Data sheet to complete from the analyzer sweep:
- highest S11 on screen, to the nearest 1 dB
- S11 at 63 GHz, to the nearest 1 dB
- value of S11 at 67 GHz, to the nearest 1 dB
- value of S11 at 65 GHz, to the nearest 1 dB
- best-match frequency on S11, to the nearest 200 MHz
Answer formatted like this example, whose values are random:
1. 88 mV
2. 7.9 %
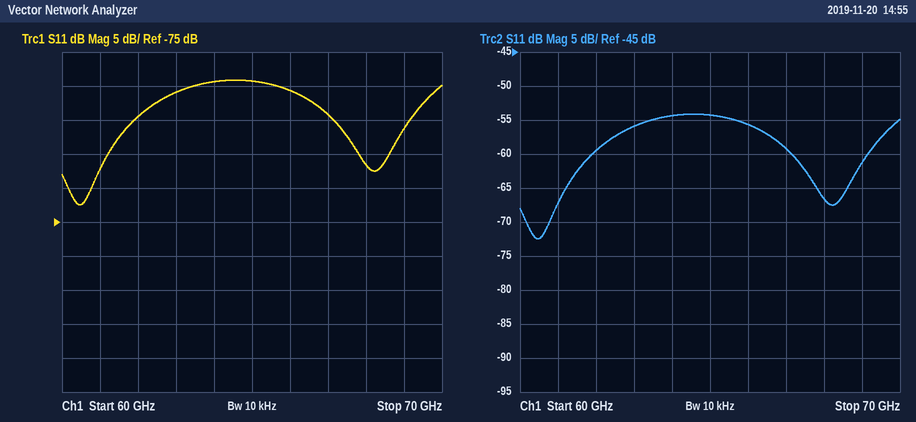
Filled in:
1. -54 dB
2. -56 dB
3. -59 dB
4. -54 dB
5. 60.4 GHz
